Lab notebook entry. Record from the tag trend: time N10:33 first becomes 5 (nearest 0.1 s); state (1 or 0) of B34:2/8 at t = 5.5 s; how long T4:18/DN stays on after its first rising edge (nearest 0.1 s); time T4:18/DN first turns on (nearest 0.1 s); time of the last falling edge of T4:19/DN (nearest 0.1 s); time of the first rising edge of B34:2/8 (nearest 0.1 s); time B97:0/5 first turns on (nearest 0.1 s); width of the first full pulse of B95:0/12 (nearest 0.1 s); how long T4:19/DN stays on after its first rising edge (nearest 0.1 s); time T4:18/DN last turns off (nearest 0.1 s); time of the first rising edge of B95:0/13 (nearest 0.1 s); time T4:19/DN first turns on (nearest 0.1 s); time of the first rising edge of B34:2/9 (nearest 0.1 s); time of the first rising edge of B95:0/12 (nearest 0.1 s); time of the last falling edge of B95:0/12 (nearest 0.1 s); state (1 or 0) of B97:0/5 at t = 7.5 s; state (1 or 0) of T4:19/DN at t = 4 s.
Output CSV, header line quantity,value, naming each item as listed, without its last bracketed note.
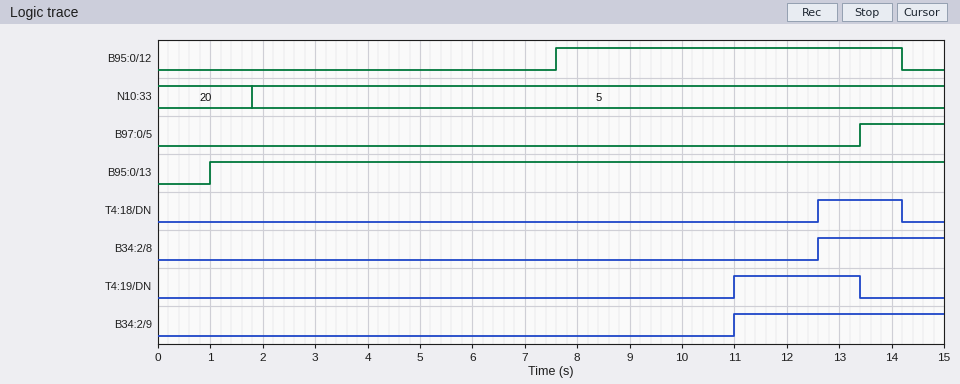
quantity,value
time N10:33 first becomes 5,1.8 s
state (1 or 0) of B34:2/8 at t = 5.5 s,0
how long T4:18/DN stays on after its first rising edge,1.6 s
time T4:18/DN first turns on,12.6 s
time of the last falling edge of T4:19/DN,13.4 s
time of the first rising edge of B34:2/8,12.6 s
time B97:0/5 first turns on,13.4 s
width of the first full pulse of B95:0/12,6.6 s
how long T4:19/DN stays on after its first rising edge,2.4 s
time T4:18/DN last turns off,14.2 s
time of the first rising edge of B95:0/13,1.0 s
time T4:19/DN first turns on,11.0 s
time of the first rising edge of B34:2/9,11.0 s
time of the first rising edge of B95:0/12,7.6 s
time of the last falling edge of B95:0/12,14.2 s
state (1 or 0) of B97:0/5 at t = 7.5 s,0
state (1 or 0) of T4:19/DN at t = 4 s,0
